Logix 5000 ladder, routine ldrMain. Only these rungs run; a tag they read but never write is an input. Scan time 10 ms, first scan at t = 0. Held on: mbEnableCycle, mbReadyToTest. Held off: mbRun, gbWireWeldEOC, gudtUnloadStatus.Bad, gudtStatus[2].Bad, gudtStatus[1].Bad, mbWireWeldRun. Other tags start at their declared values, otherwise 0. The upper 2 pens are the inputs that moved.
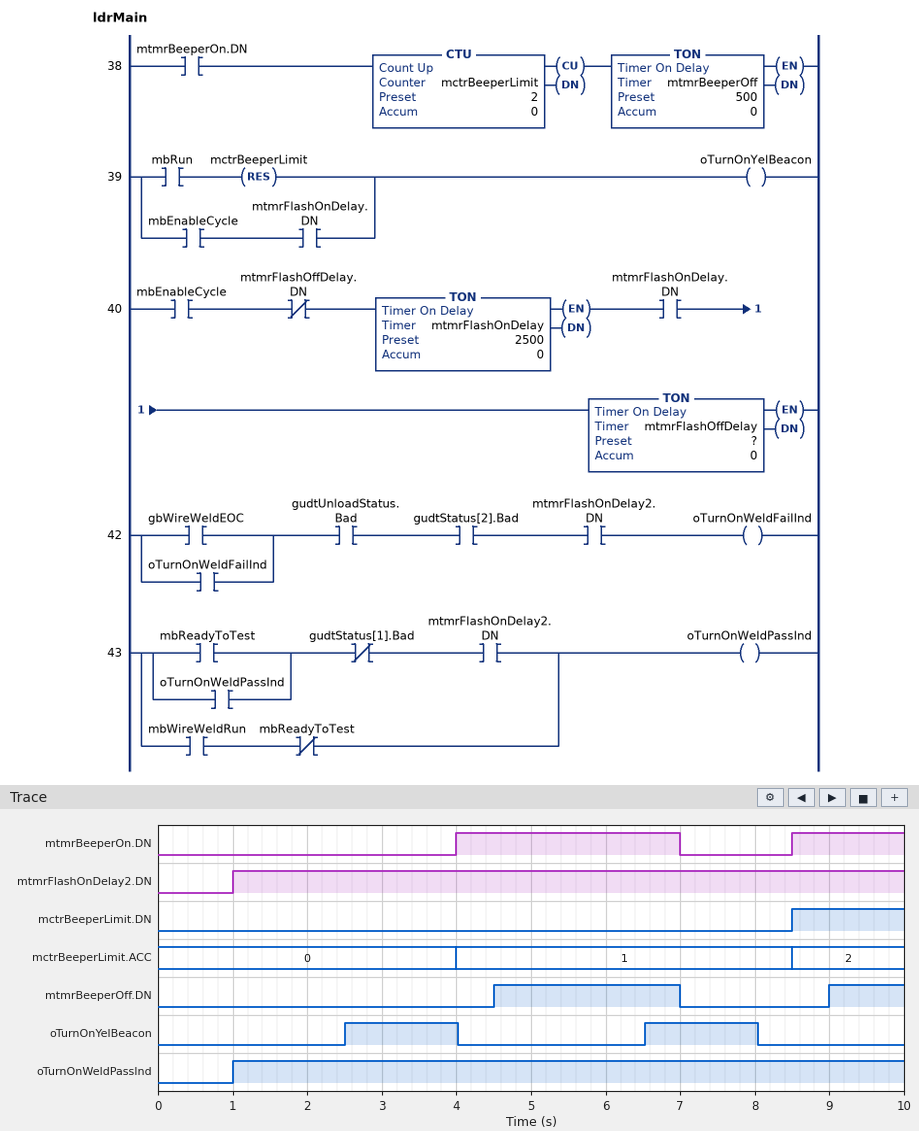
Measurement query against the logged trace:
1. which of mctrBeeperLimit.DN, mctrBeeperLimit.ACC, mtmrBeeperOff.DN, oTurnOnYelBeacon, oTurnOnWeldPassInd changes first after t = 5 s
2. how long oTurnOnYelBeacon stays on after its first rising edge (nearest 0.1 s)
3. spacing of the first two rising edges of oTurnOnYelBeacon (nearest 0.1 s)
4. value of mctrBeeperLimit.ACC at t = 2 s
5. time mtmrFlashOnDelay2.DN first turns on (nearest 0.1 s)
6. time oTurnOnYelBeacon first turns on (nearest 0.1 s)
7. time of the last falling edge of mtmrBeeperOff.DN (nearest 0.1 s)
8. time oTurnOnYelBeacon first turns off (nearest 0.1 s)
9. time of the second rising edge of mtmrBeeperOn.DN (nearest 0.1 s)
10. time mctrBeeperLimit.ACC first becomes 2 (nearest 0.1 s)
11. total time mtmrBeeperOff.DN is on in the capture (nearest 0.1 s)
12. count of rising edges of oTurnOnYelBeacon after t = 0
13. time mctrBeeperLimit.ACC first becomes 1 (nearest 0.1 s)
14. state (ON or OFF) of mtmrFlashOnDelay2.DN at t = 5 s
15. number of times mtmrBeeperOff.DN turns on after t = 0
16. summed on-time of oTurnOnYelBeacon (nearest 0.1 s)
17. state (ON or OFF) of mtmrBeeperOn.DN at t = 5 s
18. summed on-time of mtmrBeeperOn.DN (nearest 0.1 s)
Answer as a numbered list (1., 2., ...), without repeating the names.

1. oTurnOnYelBeacon
2. 1.5 s
3. 4.0 s
4. 0
5. 1.0 s
6. 2.5 s
7. 7.0 s
8. 4.0 s
9. 8.5 s
10. 8.5 s
11. 3.5 s
12. 2
13. 4.0 s
14. ON
15. 2
16. 3.0 s
17. ON
18. 4.5 s
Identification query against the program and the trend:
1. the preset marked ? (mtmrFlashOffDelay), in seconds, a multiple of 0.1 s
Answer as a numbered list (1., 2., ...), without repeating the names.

1. 1.5 s
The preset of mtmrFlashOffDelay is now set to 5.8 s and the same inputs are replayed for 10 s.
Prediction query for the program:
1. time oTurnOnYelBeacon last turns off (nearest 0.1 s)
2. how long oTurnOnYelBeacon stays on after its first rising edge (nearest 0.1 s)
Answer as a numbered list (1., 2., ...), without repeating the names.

1. 8.3 s
2. 5.8 s
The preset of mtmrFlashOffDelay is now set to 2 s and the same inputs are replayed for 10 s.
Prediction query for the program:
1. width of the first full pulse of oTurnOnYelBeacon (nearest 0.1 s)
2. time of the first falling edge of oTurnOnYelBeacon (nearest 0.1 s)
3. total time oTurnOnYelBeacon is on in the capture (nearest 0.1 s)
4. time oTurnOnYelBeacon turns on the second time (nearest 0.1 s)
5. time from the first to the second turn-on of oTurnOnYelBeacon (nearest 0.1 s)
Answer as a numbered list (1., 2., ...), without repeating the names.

1. 2.0 s
2. 4.5 s
3. 4.0 s
4. 7.0 s
5. 4.5 s
